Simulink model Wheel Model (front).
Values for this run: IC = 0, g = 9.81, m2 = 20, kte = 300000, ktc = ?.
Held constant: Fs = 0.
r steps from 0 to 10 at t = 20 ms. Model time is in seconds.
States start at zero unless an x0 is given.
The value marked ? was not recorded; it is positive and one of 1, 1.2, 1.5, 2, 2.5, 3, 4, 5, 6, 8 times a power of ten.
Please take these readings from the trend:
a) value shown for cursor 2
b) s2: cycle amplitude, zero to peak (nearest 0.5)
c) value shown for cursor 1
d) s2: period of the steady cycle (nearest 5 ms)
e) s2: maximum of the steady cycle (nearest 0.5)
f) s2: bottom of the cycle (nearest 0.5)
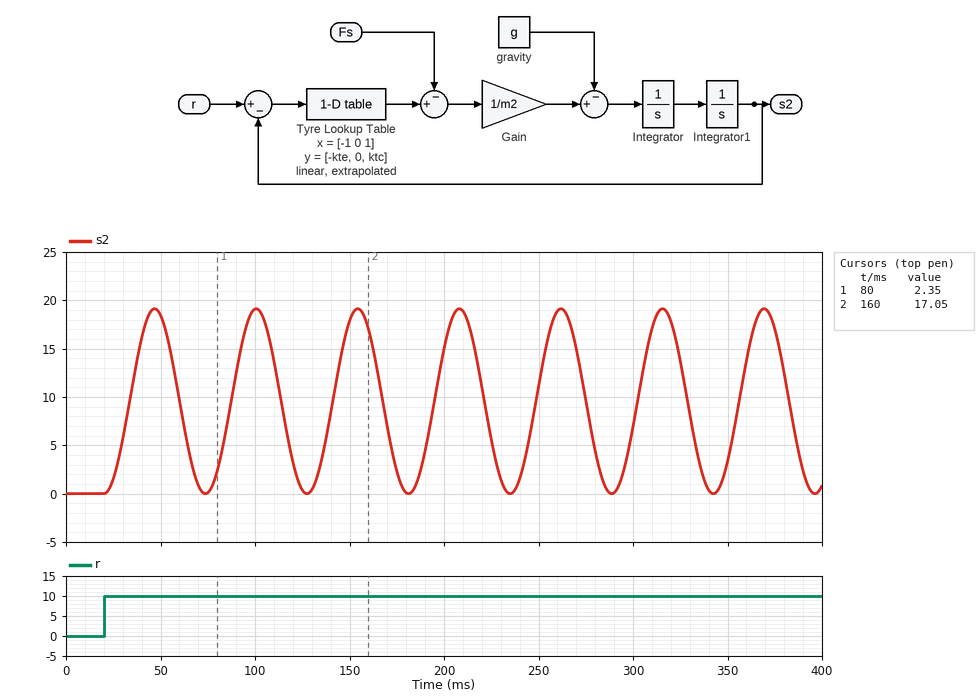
17.05
9.5
2.35
55 ms
19.0
0.0
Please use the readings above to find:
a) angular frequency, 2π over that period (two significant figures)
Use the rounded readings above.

0.11 rad/ms
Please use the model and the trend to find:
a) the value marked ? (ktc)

250000
